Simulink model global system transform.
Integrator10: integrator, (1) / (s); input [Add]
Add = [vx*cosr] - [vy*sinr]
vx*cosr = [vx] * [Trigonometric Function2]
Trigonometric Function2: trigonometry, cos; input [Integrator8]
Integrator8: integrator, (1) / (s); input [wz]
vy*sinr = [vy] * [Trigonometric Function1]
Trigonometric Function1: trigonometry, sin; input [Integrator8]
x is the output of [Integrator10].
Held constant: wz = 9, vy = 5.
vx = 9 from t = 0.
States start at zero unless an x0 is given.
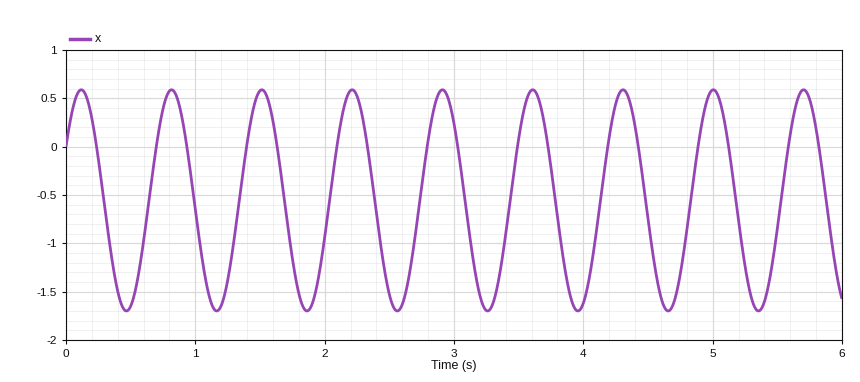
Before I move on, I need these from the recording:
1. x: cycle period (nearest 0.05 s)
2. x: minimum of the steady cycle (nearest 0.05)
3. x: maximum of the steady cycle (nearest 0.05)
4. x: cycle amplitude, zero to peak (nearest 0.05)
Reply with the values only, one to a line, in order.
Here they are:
0.70 s
-1.70
0.60
1.15
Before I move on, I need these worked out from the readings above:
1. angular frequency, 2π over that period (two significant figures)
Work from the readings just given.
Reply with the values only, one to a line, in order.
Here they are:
9.0 rad/s
